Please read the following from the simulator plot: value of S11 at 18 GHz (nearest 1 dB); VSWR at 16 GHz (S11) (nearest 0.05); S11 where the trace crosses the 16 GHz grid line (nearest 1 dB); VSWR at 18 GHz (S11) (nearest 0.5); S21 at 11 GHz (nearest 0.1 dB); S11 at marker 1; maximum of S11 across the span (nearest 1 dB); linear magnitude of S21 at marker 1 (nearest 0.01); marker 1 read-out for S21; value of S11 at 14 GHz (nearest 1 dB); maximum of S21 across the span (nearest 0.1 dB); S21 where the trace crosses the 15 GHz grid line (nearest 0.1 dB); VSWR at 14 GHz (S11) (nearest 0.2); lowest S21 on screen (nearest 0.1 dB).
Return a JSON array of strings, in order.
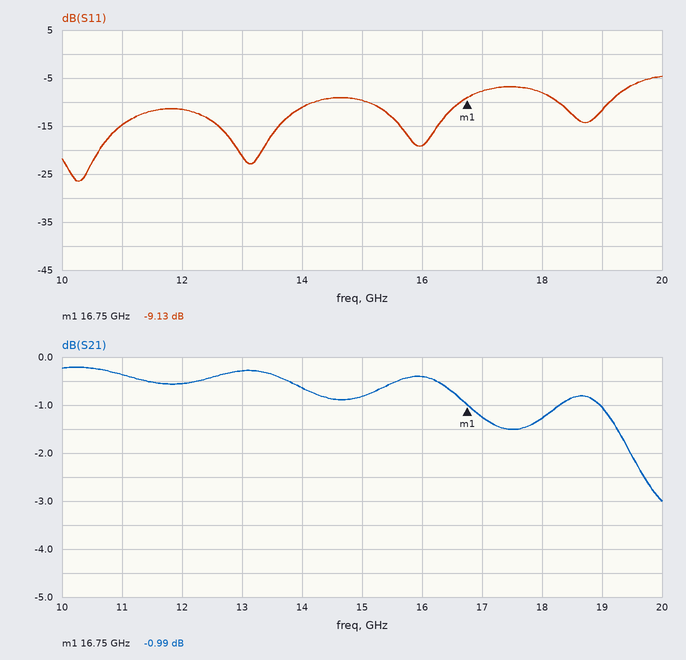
["-8 dB", "1.25", "-19 dB", "2.5", "-0.4 dB", "-9.13 dB", "-5 dB", "0.89", "-0.99 dB", "-11 dB", "-0.2 dB", "-0.8 dB", "1.8", "-3.0 dB"]
